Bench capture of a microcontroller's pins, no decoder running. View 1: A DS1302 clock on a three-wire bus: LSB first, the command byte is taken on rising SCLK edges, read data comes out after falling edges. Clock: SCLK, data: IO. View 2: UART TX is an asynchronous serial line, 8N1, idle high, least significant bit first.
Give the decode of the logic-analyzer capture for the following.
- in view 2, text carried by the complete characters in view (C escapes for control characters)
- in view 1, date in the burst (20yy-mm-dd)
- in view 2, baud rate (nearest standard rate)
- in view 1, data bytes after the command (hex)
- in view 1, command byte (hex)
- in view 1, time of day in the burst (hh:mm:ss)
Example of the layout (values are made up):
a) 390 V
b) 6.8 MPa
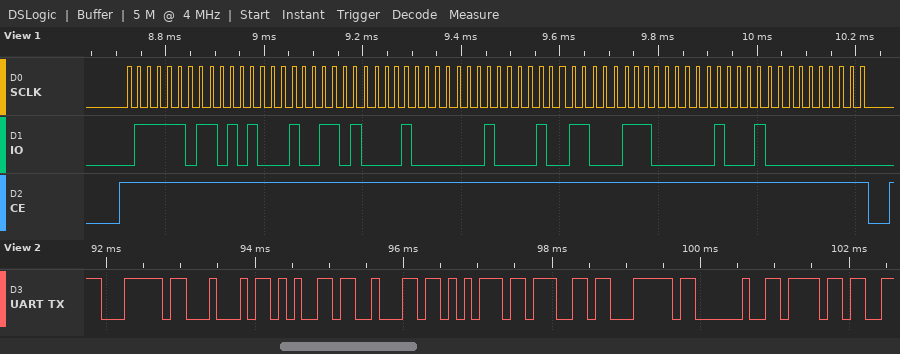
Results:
a) "|Debug| o"
b) 2022-19-08
c) 9600 baud
d) 15 59 08 08 19 07 22 00
e) 0xBE
f) 08:59:15
